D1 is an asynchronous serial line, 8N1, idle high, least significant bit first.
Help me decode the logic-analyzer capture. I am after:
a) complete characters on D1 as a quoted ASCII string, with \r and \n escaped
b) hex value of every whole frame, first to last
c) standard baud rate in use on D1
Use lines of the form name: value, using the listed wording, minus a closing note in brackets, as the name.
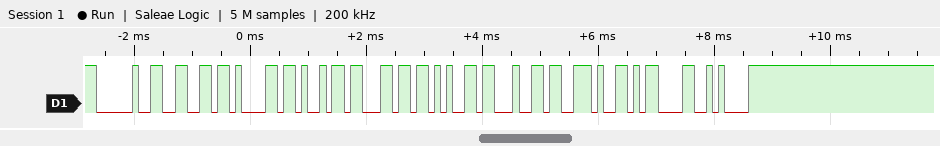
complete characters on D1 as a quoted ASCII string, with \r and \n escaped: " failed.\r\n"
hex value of every whole frame, first to last: 20 66 61 69 6C 65 64 2E 0D 0A
standard baud rate in use on D1: 9600 baud
